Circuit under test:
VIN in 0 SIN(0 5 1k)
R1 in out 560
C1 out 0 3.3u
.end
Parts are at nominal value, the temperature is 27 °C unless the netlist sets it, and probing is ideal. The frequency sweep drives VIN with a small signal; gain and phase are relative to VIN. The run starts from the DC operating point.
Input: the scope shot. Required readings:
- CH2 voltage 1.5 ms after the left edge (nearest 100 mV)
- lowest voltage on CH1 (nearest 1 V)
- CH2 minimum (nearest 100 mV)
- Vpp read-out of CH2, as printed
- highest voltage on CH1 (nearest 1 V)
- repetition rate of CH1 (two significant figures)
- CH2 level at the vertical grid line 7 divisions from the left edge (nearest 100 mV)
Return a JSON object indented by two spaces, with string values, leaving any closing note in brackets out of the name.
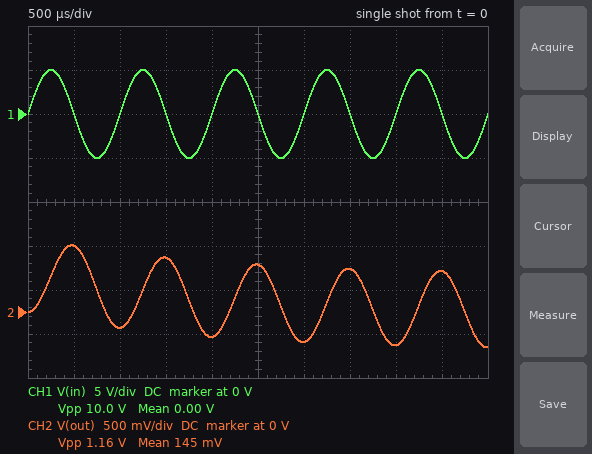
{
  "CH2 voltage 1.5 ms after the left edge": "600 mV",
  "lowest voltage on CH1": "-5 V",
  "CH2 minimum": "-400 mV",
  "Vpp read-out of CH2, as printed": "1.16 V",
  "highest voltage on CH1": "5 V",
  "repetition rate of CH1": "1.0 kHz",
  "CH2 level at the vertical grid line 7 divisions from the left edge": "500 mV"
}
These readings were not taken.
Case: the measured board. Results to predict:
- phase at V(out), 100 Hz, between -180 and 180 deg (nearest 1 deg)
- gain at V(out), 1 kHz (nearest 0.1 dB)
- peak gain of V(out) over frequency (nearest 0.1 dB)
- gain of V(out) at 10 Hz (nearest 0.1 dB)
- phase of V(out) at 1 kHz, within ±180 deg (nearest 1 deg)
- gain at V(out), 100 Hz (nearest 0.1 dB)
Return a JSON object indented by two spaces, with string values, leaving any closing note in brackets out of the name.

{
  "phase at V(out), 100 Hz, between -180 and 180 deg": "-49 deg",
  "gain at V(out), 1 kHz": "-21.3 dB",
  "peak gain of V(out) over frequency": "0 dB",
  "gain of V(out) at 10 Hz": "-0.1 dB",
  "phase of V(out) at 1 kHz, within ±180 deg": "-85 deg",
  "gain at V(out), 100 Hz": "-3.7 dB"
}
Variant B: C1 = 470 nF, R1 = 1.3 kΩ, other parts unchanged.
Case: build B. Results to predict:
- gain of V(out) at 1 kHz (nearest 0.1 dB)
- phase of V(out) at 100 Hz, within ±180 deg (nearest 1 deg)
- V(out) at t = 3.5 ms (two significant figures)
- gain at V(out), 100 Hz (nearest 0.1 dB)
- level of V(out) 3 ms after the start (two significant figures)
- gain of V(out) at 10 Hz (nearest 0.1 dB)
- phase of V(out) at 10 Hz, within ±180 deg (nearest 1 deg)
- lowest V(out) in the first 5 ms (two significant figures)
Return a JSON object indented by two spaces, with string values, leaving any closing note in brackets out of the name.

{
  "gain of V(out) at 1 kHz": "-12.0 dB",
  "phase of V(out) at 100 Hz, within ±180 deg": "-21 deg",
  "V(out) at t = 3.5 ms": "1.2 V",
  "gain at V(out), 100 Hz": "-0.6 dB",
  "level of V(out) 3 ms after the start": "-1.2 V",
  "gain of V(out) at 10 Hz": "0 dB",
  "phase of V(out) at 10 Hz, within ±180 deg": "-2 deg",
  "lowest V(out) in the first 5 ms": "-1.3 V"
}
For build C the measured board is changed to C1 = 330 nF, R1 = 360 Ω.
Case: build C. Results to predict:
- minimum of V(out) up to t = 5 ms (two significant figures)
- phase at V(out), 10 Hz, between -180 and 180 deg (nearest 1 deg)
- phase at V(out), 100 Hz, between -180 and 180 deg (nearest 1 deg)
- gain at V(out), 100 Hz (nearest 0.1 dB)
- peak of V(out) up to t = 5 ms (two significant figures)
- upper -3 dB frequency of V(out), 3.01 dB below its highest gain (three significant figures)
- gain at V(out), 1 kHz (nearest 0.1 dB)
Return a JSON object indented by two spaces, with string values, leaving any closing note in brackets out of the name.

{
  "minimum of V(out) up to t = 5 ms": "-4.0 V",
  "phase at V(out), 10 Hz, between -180 and 180 deg": "0 deg",
  "phase at V(out), 100 Hz, between -180 and 180 deg": "-4 deg",
  "gain at V(out), 100 Hz": "0 dB",
  "peak of V(out) up to t = 5 ms": "4.1 V",
  "upper -3 dB frequency of V(out), 3.01 dB below its highest gain": "1.34 kHz",
  "gain at V(out), 1 kHz": "-1.9 dB"
}
